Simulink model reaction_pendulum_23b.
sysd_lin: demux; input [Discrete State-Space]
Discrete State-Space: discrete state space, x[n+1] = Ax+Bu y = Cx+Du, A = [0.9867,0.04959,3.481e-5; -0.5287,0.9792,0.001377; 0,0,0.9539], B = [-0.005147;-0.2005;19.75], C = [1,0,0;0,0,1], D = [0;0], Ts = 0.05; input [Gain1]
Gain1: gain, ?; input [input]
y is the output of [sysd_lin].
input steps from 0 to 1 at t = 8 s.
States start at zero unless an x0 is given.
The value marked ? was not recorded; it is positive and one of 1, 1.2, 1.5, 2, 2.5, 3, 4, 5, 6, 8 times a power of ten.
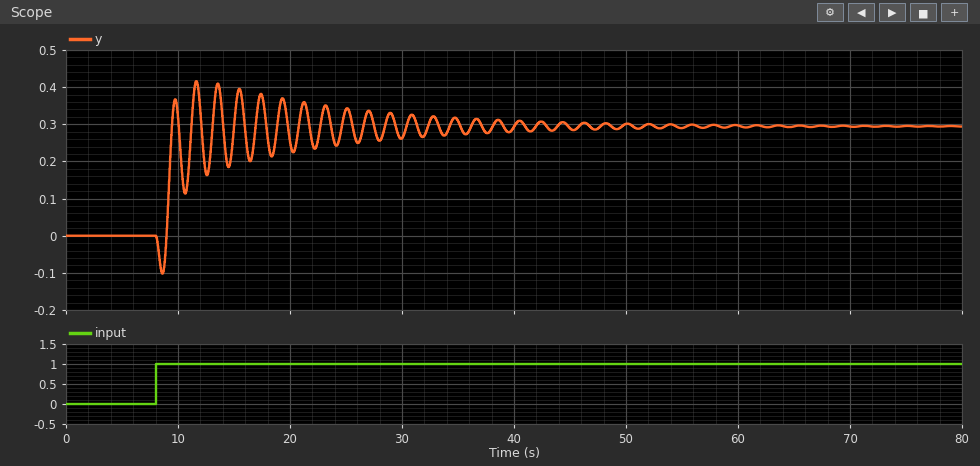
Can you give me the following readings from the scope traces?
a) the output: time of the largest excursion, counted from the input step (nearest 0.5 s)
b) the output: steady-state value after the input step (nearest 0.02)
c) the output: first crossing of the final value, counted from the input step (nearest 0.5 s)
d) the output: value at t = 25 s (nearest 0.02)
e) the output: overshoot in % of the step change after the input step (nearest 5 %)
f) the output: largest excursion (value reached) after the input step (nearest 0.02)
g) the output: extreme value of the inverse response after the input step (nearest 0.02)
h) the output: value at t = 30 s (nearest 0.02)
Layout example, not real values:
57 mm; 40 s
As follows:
3.5 s; 0.30; 1.5 s; 0.34; 40 %; 0.42; -0.10; 0.26
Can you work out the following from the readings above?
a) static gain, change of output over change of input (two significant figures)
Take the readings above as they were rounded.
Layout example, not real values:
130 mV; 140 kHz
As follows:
0.30
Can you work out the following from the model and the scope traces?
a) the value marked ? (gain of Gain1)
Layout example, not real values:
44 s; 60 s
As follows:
0.4
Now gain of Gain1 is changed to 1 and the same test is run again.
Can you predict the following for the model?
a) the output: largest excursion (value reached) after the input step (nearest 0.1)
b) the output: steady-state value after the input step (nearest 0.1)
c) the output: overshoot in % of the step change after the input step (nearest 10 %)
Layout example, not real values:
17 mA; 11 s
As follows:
1.0; 0.7; 40 %
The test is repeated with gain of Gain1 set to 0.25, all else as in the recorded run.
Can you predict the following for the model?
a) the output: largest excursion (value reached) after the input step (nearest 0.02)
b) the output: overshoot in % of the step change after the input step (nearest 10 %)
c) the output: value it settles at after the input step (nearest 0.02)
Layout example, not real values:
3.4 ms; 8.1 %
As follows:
0.26; 40 %; 0.18
